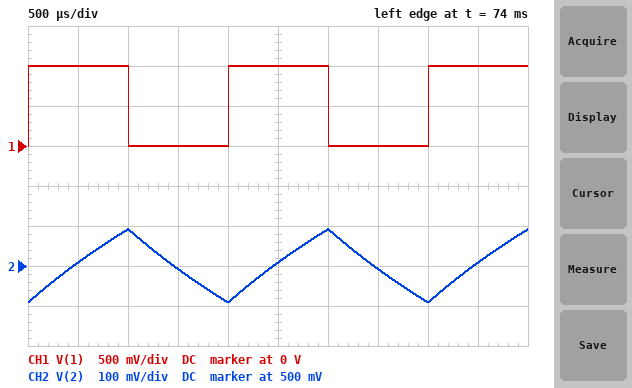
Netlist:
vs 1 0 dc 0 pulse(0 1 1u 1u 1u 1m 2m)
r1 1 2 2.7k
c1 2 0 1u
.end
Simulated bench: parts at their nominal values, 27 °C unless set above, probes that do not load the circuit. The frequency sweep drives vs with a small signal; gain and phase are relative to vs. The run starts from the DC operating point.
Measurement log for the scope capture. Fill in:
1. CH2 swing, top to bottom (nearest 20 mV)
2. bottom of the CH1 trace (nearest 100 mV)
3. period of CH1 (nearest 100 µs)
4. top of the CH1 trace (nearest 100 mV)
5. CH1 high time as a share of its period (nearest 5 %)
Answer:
180 mV
0 V
2.0 ms
1.0 V
50 %
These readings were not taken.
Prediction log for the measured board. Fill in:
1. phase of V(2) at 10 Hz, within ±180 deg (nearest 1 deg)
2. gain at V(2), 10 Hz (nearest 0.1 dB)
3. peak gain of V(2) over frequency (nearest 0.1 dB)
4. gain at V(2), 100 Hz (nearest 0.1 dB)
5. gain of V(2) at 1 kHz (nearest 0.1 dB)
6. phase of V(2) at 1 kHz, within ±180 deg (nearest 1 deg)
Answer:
-10 deg
-0.1 dB
0 dB
-5.9 dB
-24.6 dB
-87 deg
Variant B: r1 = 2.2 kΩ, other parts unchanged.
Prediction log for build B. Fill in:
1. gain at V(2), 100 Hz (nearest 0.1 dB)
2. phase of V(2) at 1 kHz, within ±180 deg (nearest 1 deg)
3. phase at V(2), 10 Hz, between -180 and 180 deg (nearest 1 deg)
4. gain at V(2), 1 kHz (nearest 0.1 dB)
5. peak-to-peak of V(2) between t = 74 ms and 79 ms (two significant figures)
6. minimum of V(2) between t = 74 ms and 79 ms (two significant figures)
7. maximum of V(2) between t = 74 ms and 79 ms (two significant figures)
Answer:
-4.6 dB
-86 deg
-8 deg
-22.8 dB
220 mV
390 mV
610 mV
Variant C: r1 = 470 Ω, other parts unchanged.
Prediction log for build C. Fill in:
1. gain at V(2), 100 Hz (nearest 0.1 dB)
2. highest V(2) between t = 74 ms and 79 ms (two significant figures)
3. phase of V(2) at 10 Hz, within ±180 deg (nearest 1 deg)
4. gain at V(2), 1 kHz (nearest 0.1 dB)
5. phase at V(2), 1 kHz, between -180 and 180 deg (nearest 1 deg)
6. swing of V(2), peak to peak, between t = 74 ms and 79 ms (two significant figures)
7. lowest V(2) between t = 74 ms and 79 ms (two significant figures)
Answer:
-0.4 dB
890 mV
-2 deg
-9.9 dB
-71 deg
790 mV
110 mV
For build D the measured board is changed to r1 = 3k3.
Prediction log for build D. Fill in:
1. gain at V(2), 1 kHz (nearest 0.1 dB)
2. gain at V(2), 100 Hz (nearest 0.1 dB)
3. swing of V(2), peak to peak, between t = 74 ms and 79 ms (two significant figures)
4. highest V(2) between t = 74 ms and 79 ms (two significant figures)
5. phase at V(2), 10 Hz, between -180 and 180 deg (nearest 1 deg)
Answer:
-26.3 dB
-7.2 dB
150 mV
580 mV
-12 deg
